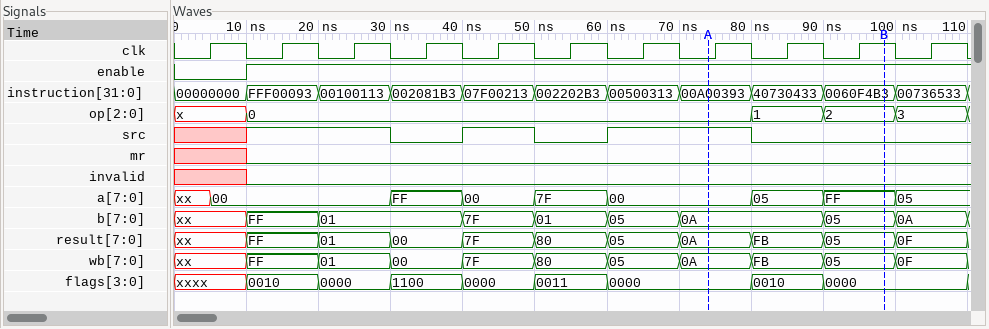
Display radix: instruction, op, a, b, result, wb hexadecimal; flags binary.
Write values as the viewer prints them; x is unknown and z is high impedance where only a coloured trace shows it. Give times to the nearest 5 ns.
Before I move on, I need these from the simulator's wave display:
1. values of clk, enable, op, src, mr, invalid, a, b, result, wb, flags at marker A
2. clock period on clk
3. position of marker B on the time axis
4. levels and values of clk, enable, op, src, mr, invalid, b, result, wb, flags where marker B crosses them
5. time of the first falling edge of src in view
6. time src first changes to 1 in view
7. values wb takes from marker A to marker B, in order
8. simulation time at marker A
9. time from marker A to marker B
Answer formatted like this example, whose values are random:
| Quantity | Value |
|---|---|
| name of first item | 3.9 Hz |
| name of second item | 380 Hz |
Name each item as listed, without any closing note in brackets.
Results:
| Quantity | Value |
|---|---|
| values of clk, enable, op, src, mr, invalid, a, b, result, wb, flags at marker A | clk=0, enable=1, op=0, src=1, mr=0, invalid=0, a=00, b=0A, result=0A, wb=0A, flags=0000 |
| clock period on clk | 10 ns |
| position of marker B on the time axis | 100 ns |
| levels and values of clk, enable, op, src, mr, invalid, b, result, wb, flags where marker B crosses them | clk=1, enable=1, op=2, src=0, mr=0, invalid=0, b=05, result=05, wb=05, flags=0000 |
| time of the first falling edge of src in view | 30 ns |
| time src first changes to 1 in view | 10 ns |
| values wb takes from marker A to marker B, in order | 0A, FB, 05 |
| simulation time at marker A | 75 ns |
| time from marker A to marker B | 25 ns |
